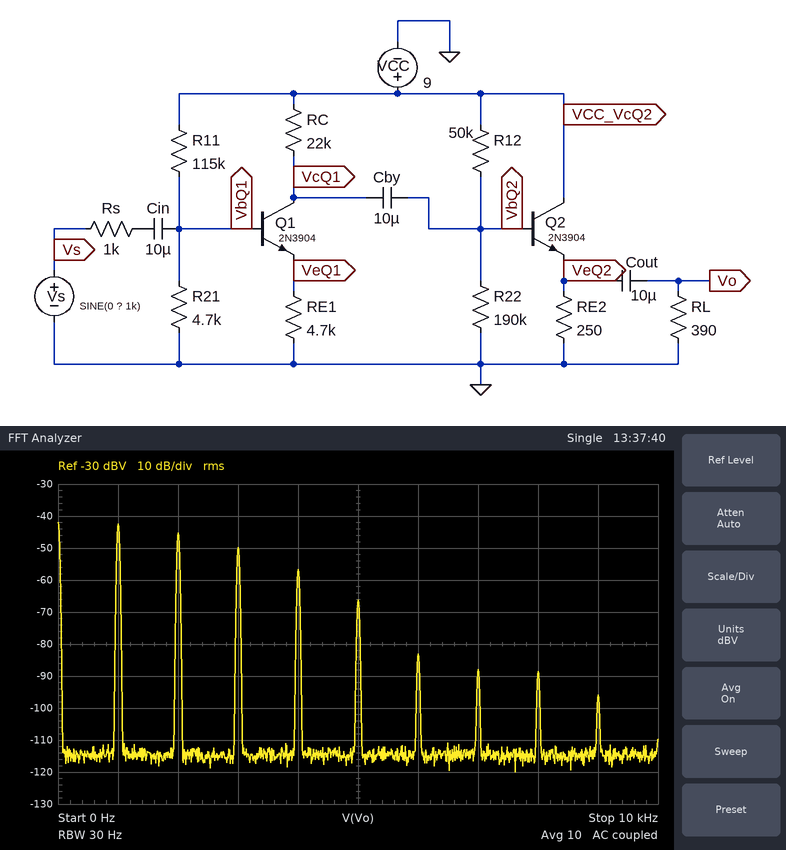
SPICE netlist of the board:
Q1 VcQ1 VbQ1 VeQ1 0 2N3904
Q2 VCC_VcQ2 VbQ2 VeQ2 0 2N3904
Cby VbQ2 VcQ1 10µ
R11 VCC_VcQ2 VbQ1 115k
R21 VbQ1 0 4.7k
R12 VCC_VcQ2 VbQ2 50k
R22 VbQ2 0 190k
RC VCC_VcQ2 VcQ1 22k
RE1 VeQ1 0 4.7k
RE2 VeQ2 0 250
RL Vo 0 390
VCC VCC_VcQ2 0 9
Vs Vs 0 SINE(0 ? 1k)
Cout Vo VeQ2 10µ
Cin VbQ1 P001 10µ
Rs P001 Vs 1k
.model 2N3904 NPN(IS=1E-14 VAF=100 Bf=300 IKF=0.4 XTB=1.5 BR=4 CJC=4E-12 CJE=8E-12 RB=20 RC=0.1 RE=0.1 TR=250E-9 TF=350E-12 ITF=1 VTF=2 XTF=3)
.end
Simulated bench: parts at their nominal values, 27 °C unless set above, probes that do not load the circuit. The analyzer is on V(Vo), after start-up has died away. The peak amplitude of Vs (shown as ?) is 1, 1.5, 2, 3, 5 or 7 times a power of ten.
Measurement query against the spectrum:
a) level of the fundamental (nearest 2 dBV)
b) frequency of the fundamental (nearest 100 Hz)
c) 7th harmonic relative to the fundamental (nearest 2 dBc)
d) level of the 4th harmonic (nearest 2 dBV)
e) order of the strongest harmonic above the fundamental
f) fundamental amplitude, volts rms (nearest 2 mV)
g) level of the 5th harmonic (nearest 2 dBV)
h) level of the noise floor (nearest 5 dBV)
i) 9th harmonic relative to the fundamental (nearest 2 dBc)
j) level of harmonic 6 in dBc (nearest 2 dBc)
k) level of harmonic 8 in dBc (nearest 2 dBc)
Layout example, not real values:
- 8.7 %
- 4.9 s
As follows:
- -42 dBV
- 1.0 kHz
- -46 dBc
- -56 dBV
- 2
- 8 mV
- -66 dBV
- -115 dBV
- -54 dBc
- -40 dBc
- -46 dBc
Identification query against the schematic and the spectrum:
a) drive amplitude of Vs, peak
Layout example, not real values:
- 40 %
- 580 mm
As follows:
- 200 mV
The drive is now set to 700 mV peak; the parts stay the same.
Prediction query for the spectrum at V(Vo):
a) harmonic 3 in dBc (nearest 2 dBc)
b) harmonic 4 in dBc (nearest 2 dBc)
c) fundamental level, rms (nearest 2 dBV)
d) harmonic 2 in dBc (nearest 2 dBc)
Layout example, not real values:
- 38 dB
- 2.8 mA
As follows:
- -14 dBc
- -30 dBc
- -12 dBV
- -4 dBc
